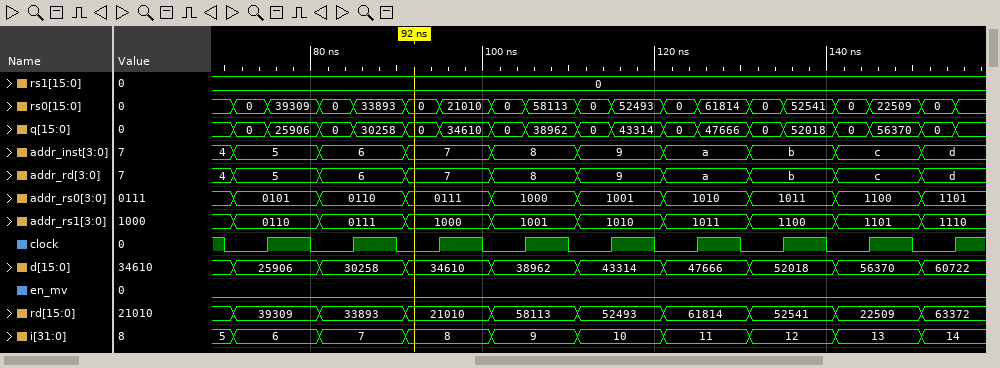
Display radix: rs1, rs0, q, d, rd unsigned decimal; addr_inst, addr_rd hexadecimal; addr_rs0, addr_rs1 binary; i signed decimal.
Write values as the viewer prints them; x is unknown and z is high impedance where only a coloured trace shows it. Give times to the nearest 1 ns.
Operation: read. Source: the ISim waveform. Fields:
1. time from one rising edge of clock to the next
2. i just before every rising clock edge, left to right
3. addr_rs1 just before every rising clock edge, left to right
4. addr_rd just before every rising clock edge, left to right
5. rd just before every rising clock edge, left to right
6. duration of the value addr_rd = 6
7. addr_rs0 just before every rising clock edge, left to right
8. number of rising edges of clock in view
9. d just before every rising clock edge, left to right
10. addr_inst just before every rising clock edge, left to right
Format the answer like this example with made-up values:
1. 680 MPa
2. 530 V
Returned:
1. 10 ns
2. 6, 7, 8, 9, 10, 11, 12, 13, 14
3. 0110, 0111, 1000, 1001, 1010, 1011, 1100, 1101, 1110
4. 5, 6, 7, 8, 9, a, b, c, d
5. 39309, 33893, 21010, 58113, 52493, 61814, 52541, 22509, 63372
6. 10 ns
7. 0101, 0110, 0111, 1000, 1001, 1010, 1011, 1100, 1101
8. 9
9. 25906, 30258, 34610, 38962, 43314, 47666, 52018, 56370, 60722
10. 5, 6, 7, 8, 9, a, b, c, d
